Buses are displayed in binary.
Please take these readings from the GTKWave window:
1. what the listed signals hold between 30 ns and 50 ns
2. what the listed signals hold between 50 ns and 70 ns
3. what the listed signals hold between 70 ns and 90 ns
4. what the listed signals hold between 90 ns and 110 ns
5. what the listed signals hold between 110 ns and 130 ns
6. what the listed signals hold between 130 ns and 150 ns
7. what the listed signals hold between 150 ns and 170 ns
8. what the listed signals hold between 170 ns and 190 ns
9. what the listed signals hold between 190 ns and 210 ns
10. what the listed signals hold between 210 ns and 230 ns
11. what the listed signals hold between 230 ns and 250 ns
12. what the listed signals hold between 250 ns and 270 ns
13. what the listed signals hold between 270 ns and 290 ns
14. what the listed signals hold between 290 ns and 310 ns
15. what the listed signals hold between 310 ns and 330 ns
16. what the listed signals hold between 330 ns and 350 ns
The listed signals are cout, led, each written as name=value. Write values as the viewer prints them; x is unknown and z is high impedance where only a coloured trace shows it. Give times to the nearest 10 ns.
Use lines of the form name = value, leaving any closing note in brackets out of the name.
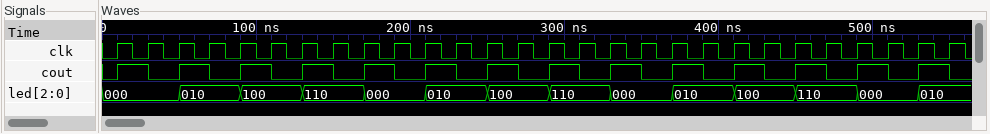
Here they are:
what the listed signals hold between 30 ns and 50 ns = cout=0, led=000
what the listed signals hold between 50 ns and 70 ns = cout=1, led=010
what the listed signals hold between 70 ns and 90 ns = cout=0, led=010
what the listed signals hold between 90 ns and 110 ns = cout=1, led=100
what the listed signals hold between 110 ns and 130 ns = cout=0, led=100
what the listed signals hold between 130 ns and 150 ns = cout=1, led=110
what the listed signals hold between 150 ns and 170 ns = cout=0, led=110
what the listed signals hold between 170 ns and 190 ns = cout=1, led=000
what the listed signals hold between 190 ns and 210 ns = cout=0, led=000
what the listed signals hold between 210 ns and 230 ns = cout=1, led=010
what the listed signals hold between 230 ns and 250 ns = cout=0, led=010
what the listed signals hold between 250 ns and 270 ns = cout=1, led=100
what the listed signals hold between 270 ns and 290 ns = cout=0, led=100
what the listed signals hold between 290 ns and 310 ns = cout=1, led=110
what the listed signals hold between 310 ns and 330 ns = cout=0, led=110
what the listed signals hold between 330 ns and 350 ns = cout=1, led=000
